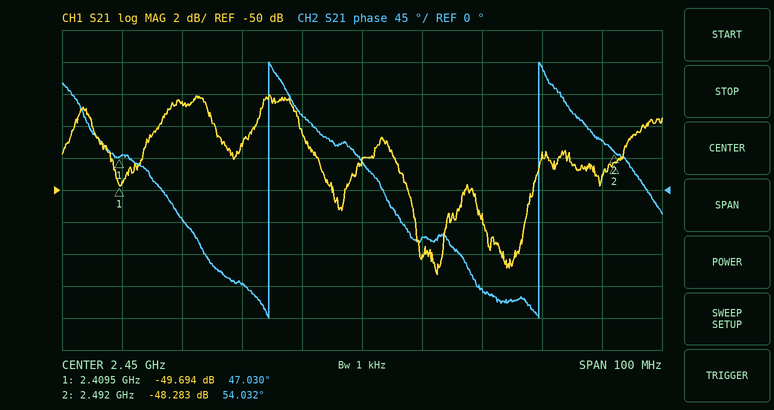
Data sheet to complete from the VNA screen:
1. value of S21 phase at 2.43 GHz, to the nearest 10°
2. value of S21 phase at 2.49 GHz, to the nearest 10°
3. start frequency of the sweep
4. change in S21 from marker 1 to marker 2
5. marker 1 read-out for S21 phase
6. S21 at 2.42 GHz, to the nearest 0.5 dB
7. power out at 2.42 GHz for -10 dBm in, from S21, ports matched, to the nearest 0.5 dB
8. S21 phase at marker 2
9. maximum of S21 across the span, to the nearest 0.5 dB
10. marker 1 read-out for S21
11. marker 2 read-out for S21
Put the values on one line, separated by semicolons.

-130°; 70°; 2.4 GHz; 1.411 dB; 47.030°; -44.5 dB; -54.5 dBm; 54.032°; -44.0 dB; -49.694 dB; -48.283 dB
